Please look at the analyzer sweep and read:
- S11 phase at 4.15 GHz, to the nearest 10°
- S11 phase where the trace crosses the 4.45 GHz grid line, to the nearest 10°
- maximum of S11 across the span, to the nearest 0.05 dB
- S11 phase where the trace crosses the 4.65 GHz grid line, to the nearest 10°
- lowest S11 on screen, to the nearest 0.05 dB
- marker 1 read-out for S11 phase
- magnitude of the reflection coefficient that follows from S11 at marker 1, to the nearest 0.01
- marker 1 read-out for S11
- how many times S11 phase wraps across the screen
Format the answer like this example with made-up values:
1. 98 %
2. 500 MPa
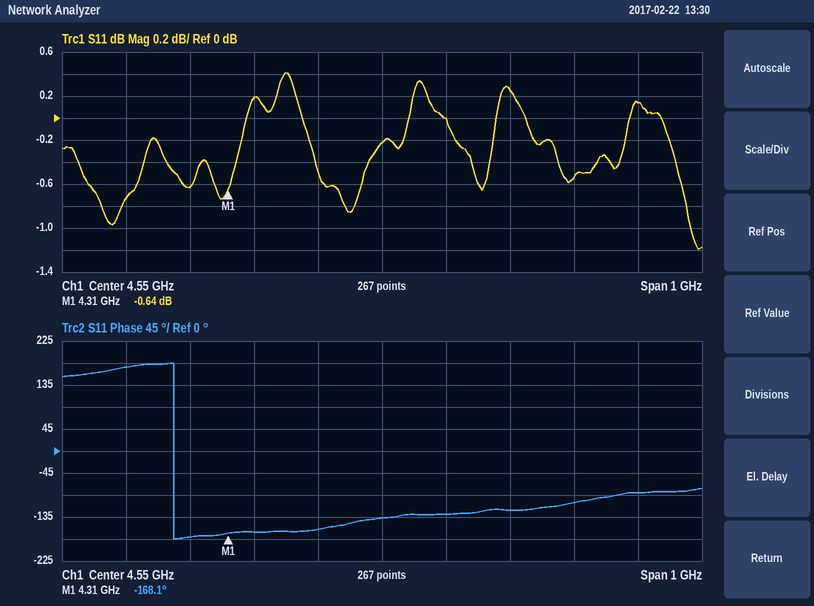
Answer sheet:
1. 170°
2. -160°
3. 0.40 dB
4. -130°
5. -1.20 dB
6. -168.1°
7. 0.93
8. -0.64 dB
9. 1
